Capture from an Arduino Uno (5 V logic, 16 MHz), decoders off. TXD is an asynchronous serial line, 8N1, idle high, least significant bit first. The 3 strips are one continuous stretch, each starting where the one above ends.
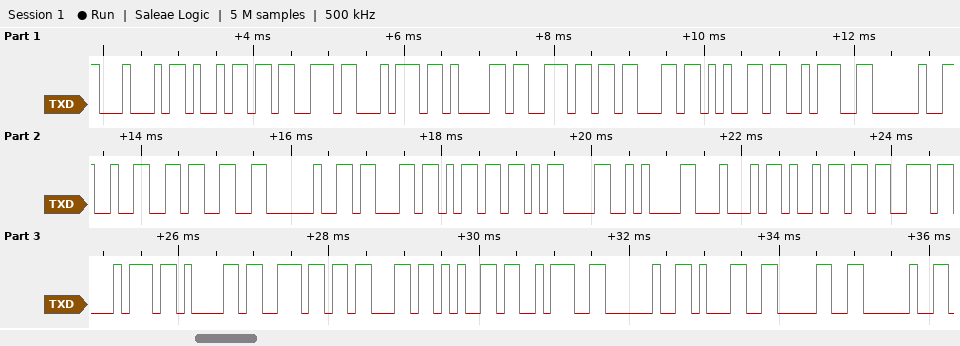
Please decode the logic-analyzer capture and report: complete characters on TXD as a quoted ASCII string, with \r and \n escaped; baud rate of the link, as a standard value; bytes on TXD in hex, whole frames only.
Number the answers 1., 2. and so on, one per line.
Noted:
1. "Distance: 23 cm\r\nDistance: 10 "
2. 9600 baud
3. 0x44 0x69 0x73 0x74 0x61 0x6E 0x63 0x65 0x3A 0x20 0x32 0x33 0x20 0x63 0x6D 0x0D 0x0A 0x44 0x69 0x73 0x74 0x61 0x6E 0x63 0x65 0x3A 0x20 0x31 0x30 0x20
